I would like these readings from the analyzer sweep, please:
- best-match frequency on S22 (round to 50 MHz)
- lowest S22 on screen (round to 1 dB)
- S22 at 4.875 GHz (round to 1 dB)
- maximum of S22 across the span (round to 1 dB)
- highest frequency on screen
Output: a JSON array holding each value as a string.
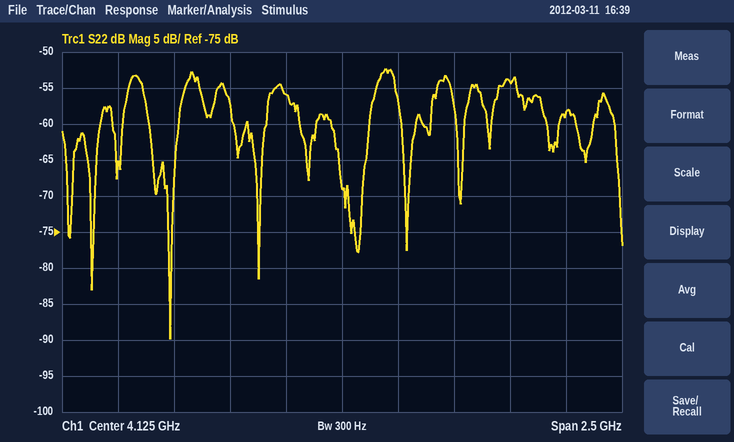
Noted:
["3.35 GHz", "-90 dB", "-54 dB", "-52 dB", "5.375 GHz"]
